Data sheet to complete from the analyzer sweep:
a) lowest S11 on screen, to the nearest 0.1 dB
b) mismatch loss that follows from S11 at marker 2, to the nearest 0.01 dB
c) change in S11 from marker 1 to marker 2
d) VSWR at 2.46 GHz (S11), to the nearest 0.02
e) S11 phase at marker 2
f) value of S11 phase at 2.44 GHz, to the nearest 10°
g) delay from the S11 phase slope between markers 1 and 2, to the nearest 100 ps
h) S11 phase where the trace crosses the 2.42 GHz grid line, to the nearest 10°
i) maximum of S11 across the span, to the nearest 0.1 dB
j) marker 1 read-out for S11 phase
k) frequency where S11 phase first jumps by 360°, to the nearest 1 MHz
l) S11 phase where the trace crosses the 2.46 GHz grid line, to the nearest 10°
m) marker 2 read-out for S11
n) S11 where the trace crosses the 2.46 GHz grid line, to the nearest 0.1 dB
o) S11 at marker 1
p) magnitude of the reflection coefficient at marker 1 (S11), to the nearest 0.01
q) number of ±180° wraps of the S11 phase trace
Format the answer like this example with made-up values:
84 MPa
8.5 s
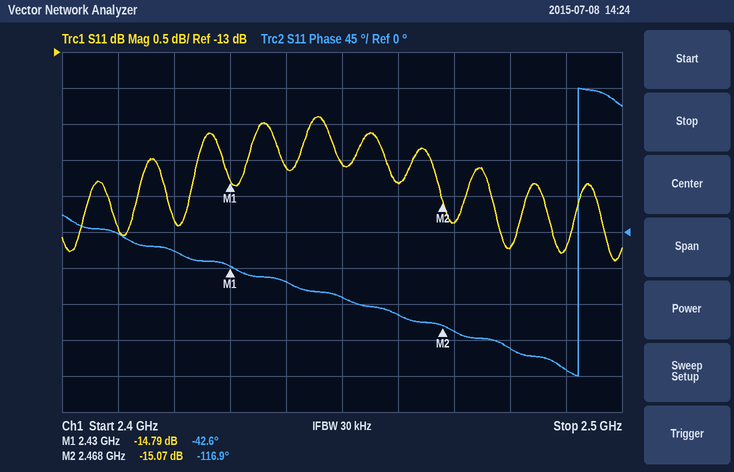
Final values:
-15.9 dB
0.14 dB
-0.28 dB
1.44
-116.9°
-60°
5.4 ns
-20°
-13.9 dB
-42.6°
2.492 GHz
-100°
-15.07 dB
-14.8 dB
-14.79 dB
0.18
1
